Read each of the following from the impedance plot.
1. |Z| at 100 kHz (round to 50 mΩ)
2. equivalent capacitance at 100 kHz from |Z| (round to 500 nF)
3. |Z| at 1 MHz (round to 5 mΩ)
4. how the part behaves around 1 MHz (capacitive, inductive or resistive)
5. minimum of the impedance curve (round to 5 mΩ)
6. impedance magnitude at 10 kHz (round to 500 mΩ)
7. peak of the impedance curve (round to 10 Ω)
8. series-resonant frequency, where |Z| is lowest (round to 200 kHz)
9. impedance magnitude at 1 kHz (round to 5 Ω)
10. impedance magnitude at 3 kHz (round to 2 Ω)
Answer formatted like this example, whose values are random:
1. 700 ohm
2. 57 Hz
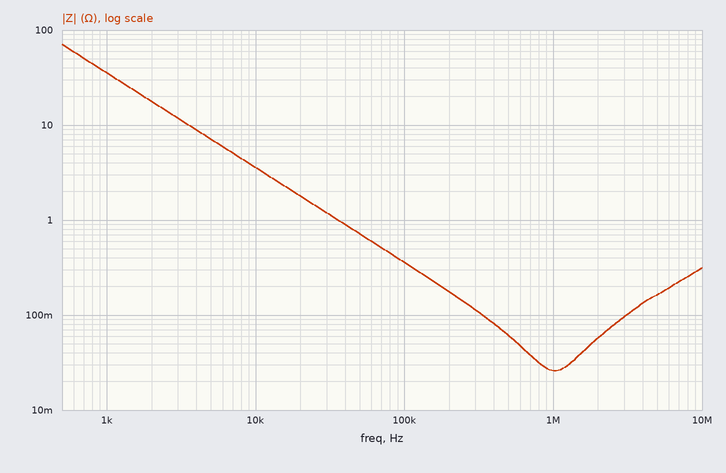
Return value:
1. 350 mΩ
2. 4.5 µF
3. 25 mΩ
4. resistive
5. 25 mΩ
6. 3.5 Ω
7. 70 Ω
8. 1.0 MHz
9. 35 Ω
10. 12 Ω
